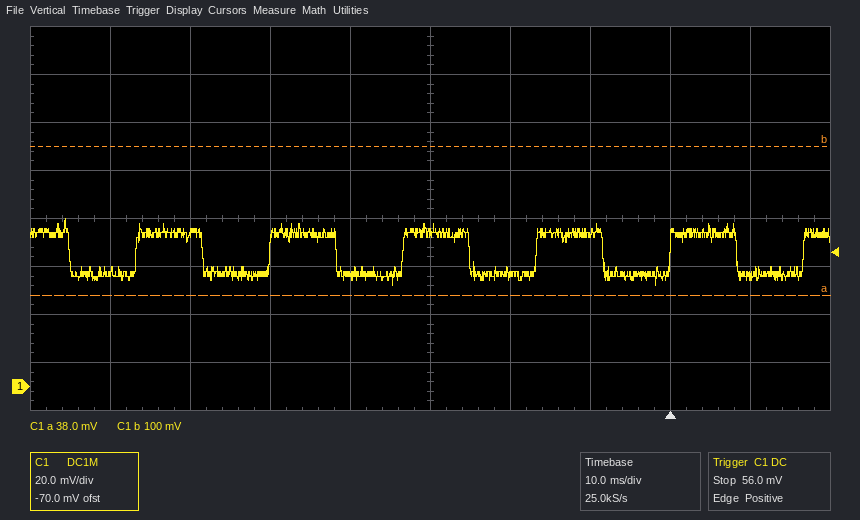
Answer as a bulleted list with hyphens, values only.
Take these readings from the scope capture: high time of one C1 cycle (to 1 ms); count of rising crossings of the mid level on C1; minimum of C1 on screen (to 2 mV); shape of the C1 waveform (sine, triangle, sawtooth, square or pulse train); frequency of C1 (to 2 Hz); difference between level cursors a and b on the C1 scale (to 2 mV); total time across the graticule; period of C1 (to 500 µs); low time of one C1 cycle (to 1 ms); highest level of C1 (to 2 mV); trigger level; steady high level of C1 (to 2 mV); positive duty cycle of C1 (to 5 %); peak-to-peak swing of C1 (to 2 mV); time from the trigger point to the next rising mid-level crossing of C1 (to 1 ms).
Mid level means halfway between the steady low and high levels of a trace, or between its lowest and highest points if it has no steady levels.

- 8 ms
- 6
- 42 mV
- square
- 60 Hz
- 62 mV
- 100 ms
- 16.5 ms
- 8 ms
- 70 mV
- 56.0 mV
- 64 mV
- 50 %
- 28 mV
- 17 ms
